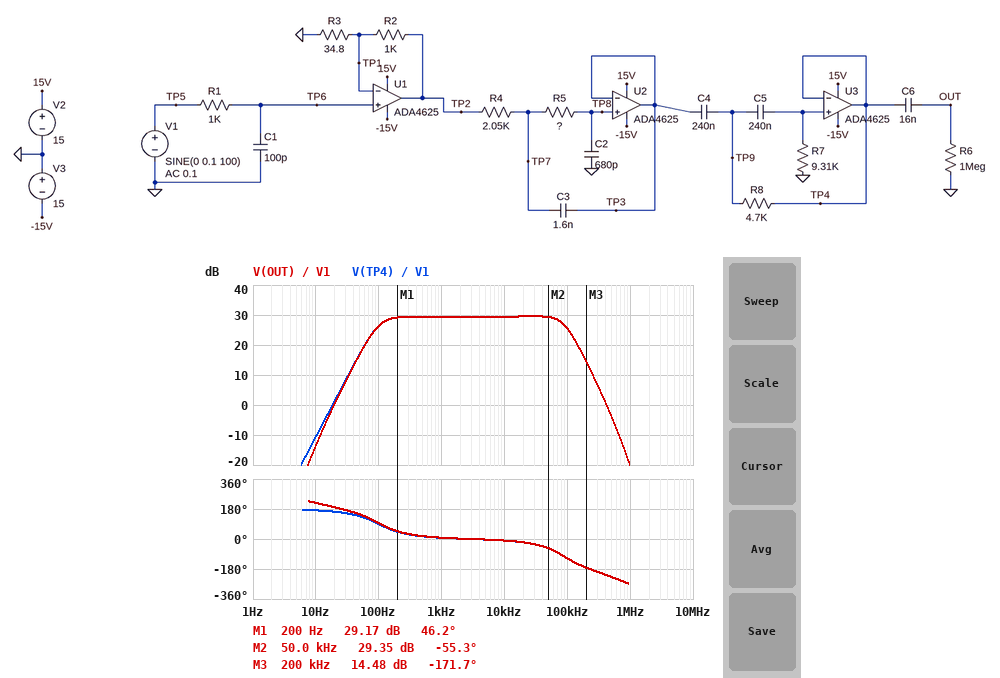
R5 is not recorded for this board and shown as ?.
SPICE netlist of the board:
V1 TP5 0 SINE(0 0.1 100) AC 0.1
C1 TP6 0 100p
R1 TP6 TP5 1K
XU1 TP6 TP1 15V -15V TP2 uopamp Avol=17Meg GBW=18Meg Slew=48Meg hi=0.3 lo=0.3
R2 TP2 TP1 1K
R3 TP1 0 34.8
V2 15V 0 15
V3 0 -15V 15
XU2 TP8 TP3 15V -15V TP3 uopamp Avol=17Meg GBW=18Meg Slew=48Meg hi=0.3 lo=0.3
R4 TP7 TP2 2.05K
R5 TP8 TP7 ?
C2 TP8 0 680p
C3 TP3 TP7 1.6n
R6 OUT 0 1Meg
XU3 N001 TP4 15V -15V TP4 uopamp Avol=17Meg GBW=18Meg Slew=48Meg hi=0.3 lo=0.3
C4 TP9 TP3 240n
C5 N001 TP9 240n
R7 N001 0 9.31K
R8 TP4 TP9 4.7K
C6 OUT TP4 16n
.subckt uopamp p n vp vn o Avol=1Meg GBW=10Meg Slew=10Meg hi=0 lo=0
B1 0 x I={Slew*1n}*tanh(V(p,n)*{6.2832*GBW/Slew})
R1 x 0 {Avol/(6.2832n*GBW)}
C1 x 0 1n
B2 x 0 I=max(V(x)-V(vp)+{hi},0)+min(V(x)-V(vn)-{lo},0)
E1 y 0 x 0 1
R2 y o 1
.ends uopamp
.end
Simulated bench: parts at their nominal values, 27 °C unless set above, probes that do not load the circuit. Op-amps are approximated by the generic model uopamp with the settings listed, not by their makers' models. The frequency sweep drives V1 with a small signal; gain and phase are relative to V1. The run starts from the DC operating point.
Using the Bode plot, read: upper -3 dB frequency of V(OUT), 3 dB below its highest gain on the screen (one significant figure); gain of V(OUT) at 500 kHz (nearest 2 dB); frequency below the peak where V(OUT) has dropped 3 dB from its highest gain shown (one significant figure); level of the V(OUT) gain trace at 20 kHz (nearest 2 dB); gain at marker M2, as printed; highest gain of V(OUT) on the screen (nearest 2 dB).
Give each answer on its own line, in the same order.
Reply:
90 kHz
-4 dB
100 Hz
30 dB
29.35 dB
30 dB
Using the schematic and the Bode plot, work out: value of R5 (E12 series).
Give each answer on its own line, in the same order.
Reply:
1.5 kΩ
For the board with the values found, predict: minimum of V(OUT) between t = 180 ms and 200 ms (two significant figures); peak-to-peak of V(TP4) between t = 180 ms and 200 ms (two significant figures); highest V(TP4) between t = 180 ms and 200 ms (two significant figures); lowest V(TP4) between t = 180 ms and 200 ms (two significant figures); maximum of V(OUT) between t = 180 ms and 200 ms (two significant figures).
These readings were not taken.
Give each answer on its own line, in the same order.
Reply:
-2.1 V
4.2 V
2.1 V
-2.1 V
2.1 V
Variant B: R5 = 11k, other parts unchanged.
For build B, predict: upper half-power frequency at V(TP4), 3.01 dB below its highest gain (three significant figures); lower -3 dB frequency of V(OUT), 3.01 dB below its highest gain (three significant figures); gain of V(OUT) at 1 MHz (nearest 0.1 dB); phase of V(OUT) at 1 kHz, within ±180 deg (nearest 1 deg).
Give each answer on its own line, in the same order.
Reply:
24.1 kHz
101 Hz
-37.5 dB
5 deg
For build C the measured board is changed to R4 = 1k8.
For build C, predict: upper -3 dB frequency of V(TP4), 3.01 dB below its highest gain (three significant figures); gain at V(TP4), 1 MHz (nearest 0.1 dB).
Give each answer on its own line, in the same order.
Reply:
97.6 kHz
-19.1 dB
